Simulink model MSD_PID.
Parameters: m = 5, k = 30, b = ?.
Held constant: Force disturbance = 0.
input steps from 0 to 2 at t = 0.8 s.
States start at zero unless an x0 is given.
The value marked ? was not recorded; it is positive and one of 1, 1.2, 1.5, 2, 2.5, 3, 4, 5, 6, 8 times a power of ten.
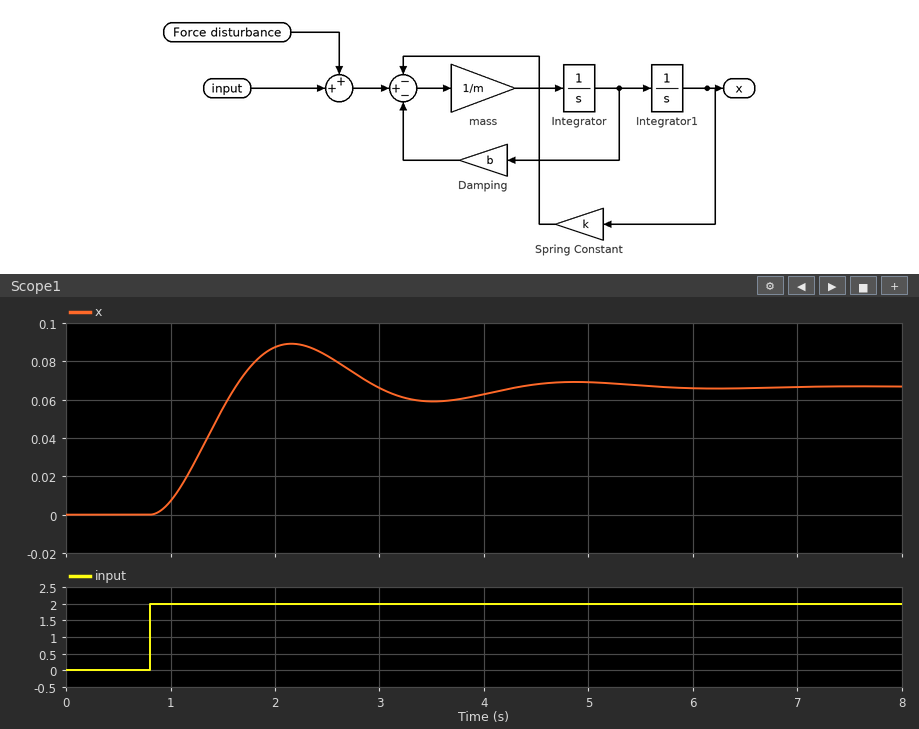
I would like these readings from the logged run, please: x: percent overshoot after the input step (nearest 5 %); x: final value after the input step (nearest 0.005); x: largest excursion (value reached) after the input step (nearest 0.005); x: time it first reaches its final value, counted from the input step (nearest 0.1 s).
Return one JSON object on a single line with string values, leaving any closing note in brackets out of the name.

{"x: percent overshoot after the input step": "35 %", "x: final value after the input step": "0.065", "x: largest excursion (value reached) after the input step": "0.090", "x: time it first reaches its final value, counted from the input step": "0.8 s"}
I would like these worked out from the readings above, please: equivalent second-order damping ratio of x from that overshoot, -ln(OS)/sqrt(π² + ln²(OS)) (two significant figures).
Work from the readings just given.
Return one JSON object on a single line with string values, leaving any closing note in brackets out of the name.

{"equivalent second-order damping ratio of x from that overshoot, -ln(OS)/sqrt(π² + ln²(OS))": "0.32"}
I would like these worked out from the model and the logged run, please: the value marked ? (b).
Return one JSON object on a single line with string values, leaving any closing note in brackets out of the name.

{"the value marked ?": "8"}
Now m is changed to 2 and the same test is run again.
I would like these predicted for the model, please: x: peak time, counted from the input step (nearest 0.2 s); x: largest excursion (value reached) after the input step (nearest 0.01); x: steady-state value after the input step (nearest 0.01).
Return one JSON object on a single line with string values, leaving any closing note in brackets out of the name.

{"x: peak time, counted from the input step": "1.0 s", "x: largest excursion (value reached) after the input step": "0.08", "x: steady-state value after the input step": "0.07"}
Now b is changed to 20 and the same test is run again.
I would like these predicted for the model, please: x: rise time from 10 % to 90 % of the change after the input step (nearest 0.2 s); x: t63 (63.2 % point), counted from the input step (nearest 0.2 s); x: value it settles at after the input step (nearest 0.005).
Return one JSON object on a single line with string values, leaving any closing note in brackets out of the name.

{"x: rise time from 10 % to 90 % of the change after the input step": "1.0 s", "x: t63 (63.2 % point), counted from the input step": "0.8 s", "x: value it settles at after the input step": "0.065"}
